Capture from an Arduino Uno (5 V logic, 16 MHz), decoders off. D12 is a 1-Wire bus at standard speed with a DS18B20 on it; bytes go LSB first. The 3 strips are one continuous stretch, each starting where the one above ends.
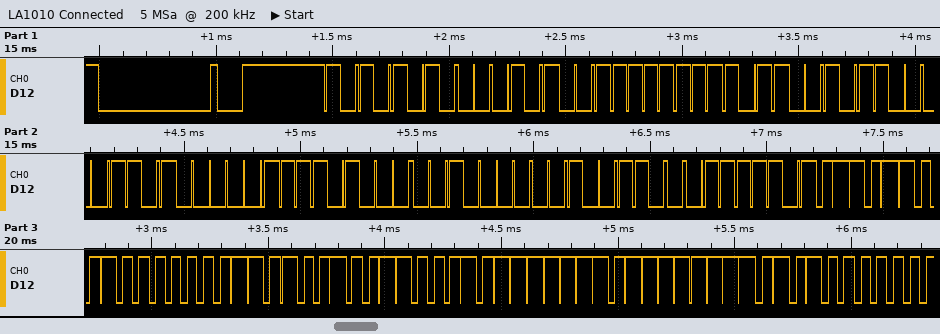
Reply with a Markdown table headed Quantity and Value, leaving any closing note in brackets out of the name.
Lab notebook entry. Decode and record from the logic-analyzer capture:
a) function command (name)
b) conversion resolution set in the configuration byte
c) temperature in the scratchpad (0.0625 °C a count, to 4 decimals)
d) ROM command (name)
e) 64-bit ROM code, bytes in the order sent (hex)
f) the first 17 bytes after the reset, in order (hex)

| Quantity | Value |
|---|---|
| function command | Read Scratchpad |
| conversion resolution set in the configuration byte | 12 bits |
| temperature in the scratchpad | 19.3750 °C |
| ROM command | Match ROM |
| 64-bit ROM code, bytes in the order sent | 28 FF 4D C3 82 17 04 32 |
| the first 17 bytes after the reset, in order | 55 28 FF 4D C3 82 17 04 32 BE 36 01 4B 46 7F FF 0A |
